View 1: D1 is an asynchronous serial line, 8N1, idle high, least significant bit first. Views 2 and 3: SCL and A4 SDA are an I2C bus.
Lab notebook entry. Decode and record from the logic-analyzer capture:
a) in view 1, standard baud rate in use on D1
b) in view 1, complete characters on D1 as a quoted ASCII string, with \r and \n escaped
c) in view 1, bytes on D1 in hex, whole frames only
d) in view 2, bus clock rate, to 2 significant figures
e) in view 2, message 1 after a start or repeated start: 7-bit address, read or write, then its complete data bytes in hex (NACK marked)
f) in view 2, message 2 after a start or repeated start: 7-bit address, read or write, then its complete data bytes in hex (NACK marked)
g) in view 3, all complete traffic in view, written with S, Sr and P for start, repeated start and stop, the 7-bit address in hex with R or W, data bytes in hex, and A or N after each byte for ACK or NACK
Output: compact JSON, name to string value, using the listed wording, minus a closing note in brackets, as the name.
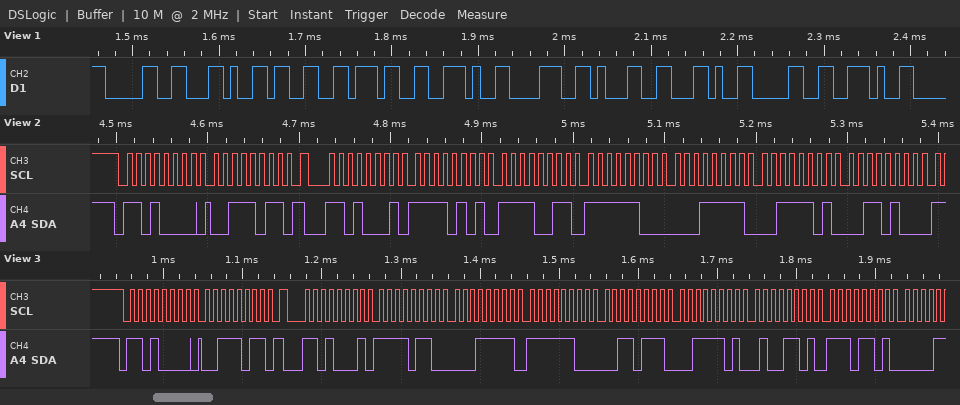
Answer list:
{"in view 1, standard baud rate in use on D1": "115200 baud", "in view 1, complete characters on D1 as a quoted ASCII string, with \\r and \\n escaped": "\"0,37.81,0.\"", "in view 1, bytes on D1 in hex, whole frames only": "30 2C 33 37 2E 38 31 2C 30 2E", "in view 2, bus clock rate, to 2 significant figures": "100 kHz", "in view 2, message 1 after a start or repeated start: 7-bit address, read or write, then its complete data bytes in hex": "0x68 write: 3B", "in view 2, message 2 after a start or repeated start: 7-bit address, read or write, then its complete data bytes in hex": "0x68 read: F5 F3 FC 1F 3D 34", "in view 3, all complete traffic in view, written with S, Sr and P for start, repeated start and stop, the 7-bit address in hex with R or W, data bytes in hex, and A or N after each byte for ACK or NACK": "S 68W A 3B A Sr 68R A F6 A 1F A FC A 37 A 3D A 4D A ED A"}
